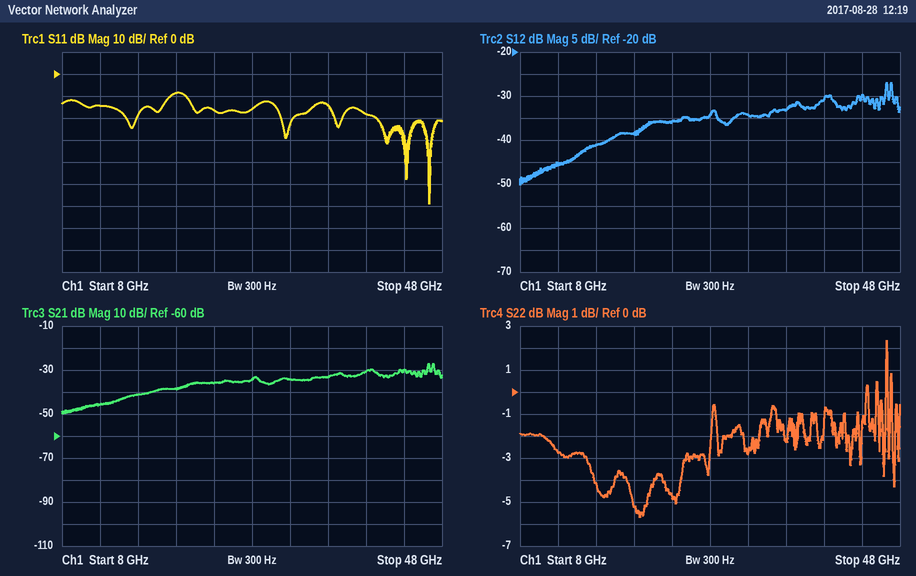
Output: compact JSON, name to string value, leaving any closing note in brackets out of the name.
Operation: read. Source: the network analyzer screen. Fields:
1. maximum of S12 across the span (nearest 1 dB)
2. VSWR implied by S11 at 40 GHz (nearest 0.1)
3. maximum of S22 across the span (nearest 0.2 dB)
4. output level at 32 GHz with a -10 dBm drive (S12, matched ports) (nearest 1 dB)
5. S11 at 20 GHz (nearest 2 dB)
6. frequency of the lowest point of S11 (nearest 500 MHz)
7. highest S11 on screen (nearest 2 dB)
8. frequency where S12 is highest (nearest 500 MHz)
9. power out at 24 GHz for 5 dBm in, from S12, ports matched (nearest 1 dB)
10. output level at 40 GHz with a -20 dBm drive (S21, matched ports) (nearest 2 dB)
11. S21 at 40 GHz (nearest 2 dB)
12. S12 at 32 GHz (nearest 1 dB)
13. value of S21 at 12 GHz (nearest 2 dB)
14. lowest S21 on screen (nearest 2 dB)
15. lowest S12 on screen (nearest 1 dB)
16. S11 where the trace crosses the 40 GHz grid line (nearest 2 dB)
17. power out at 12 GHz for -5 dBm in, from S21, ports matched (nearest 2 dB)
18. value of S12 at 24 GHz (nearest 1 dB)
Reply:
{"maximum of S12 across the span": "-27 dB", "VSWR implied by S11 at 40 GHz": "1.3", "maximum of S22 across the span": "2.4 dB", "output level at 32 GHz with a -10 dBm drive (S12, matched ports)": "-44 dBm", "S11 at 20 GHz": "-8 dB", "frequency of the lowest point of S11": "46.5 GHz", "highest S11 on screen": "-8 dB", "frequency where S12 is highest": "46.5 GHz", "power out at 24 GHz for 5 dBm in, from S12, ports matched": "-31 dBm", "output level at 40 GHz with a -20 dBm drive (S21, matched ports)": "-50 dBm", "S21 at 40 GHz": "-30 dB", "S12 at 32 GHz": "-34 dB", "value of S21 at 12 GHz": "-46 dB", "lowest S21 on screen": "-50 dB", "lowest S12 on screen": "-50 dB", "S11 where the trace crosses the 40 GHz grid line": "-18 dB", "power out at 12 GHz for -5 dBm in, from S21, ports matched": "-50 dBm", "value of S12 at 24 GHz": "-36 dB"}
